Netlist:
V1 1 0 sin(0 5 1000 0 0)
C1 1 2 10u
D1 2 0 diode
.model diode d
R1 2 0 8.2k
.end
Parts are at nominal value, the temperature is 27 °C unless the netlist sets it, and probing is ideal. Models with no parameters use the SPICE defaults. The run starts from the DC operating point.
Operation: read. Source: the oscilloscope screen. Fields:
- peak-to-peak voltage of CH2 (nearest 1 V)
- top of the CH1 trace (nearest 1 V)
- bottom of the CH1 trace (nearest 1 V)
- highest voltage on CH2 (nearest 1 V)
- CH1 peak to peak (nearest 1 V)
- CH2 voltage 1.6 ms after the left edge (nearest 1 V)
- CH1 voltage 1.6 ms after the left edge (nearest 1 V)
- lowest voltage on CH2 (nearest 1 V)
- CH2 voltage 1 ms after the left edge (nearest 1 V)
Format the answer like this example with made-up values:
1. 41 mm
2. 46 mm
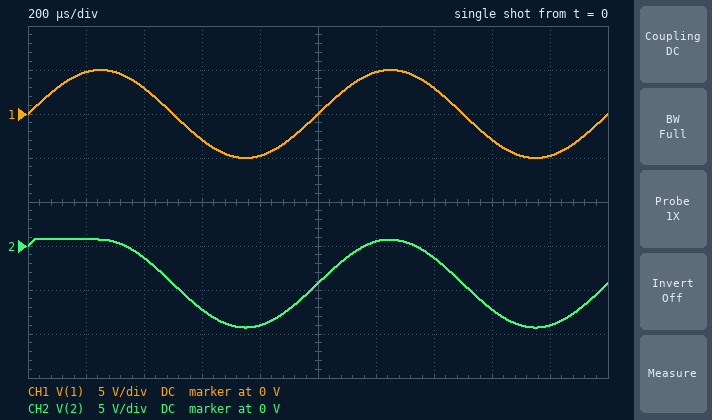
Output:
1. 10 V
2. 5 V
3. -5 V
4. 1 V
5. 10 V
6. -7 V
7. -3 V
8. -9 V
9. -4 V
